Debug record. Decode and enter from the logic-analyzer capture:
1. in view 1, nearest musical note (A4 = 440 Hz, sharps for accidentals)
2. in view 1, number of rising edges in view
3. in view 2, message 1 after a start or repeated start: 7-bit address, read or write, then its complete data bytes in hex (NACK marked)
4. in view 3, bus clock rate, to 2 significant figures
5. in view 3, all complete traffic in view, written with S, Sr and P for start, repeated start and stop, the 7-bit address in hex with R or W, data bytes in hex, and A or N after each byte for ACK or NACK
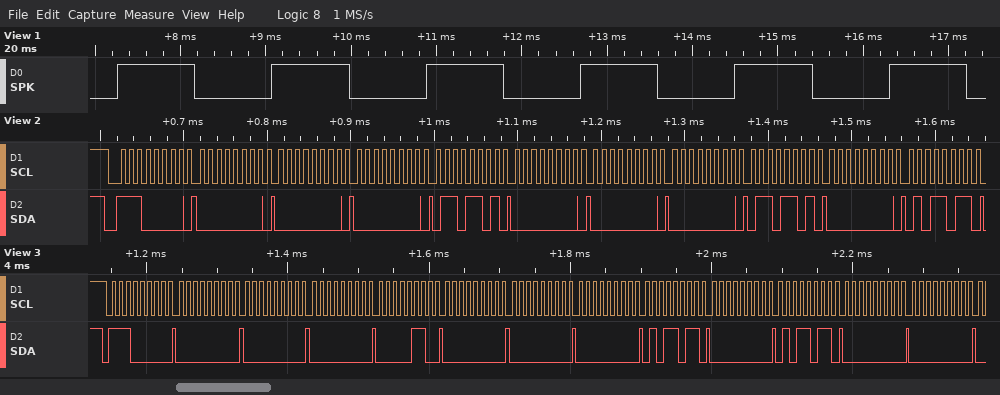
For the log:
C#5
6
0x70 write: 00 00 00 6D 00 00 00 6D 00 5B
100 kHz
S 70W A 00 A 00 A 00 A 06 A 00 A 00 A 00 A 5B A 00 A 5B A 00 A 00 A
